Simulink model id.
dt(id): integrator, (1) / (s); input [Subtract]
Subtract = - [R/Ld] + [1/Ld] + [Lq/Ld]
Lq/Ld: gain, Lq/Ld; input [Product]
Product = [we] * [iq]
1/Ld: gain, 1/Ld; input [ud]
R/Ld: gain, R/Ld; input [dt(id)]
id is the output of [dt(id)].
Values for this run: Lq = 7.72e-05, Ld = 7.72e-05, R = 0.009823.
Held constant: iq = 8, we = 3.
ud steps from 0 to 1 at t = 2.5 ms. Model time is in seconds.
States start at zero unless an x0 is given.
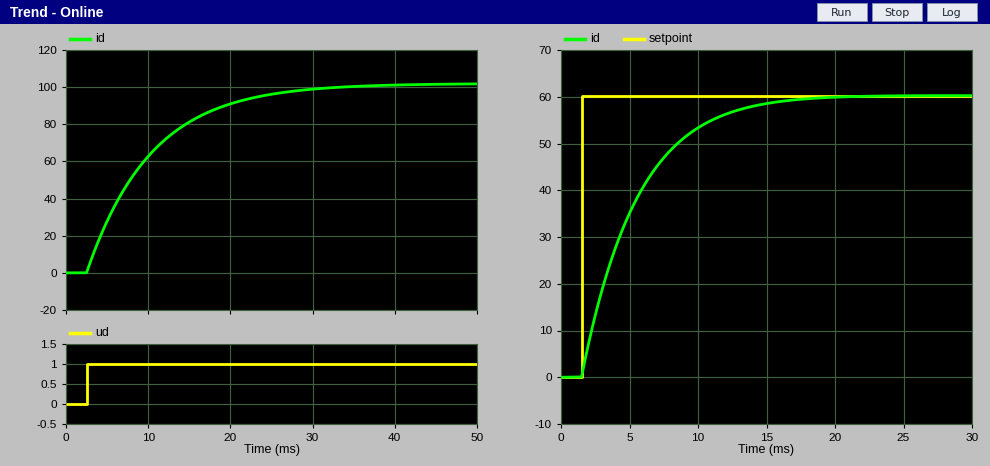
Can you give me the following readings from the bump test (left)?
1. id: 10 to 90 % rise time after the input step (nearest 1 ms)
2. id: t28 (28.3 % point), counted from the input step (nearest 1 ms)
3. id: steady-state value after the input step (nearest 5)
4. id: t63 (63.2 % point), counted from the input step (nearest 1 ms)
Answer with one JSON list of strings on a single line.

["17 ms", "3 ms", "100", "8 ms"]
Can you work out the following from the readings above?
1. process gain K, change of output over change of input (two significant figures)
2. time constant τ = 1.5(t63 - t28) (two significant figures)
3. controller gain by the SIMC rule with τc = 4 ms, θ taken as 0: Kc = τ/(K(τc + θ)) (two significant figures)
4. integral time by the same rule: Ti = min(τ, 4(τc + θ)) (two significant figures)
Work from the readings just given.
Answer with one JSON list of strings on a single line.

["100", "7.5 ms", "0.019", "7.5 ms"]
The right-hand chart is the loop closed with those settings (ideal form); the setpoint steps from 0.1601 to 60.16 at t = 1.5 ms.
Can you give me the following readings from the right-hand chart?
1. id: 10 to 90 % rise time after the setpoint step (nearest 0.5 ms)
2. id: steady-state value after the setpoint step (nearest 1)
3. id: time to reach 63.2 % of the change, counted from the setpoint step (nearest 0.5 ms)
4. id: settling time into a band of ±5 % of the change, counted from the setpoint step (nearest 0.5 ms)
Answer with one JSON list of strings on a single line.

["8.5 ms", "60", "4.0 ms", "11.5 ms"]
